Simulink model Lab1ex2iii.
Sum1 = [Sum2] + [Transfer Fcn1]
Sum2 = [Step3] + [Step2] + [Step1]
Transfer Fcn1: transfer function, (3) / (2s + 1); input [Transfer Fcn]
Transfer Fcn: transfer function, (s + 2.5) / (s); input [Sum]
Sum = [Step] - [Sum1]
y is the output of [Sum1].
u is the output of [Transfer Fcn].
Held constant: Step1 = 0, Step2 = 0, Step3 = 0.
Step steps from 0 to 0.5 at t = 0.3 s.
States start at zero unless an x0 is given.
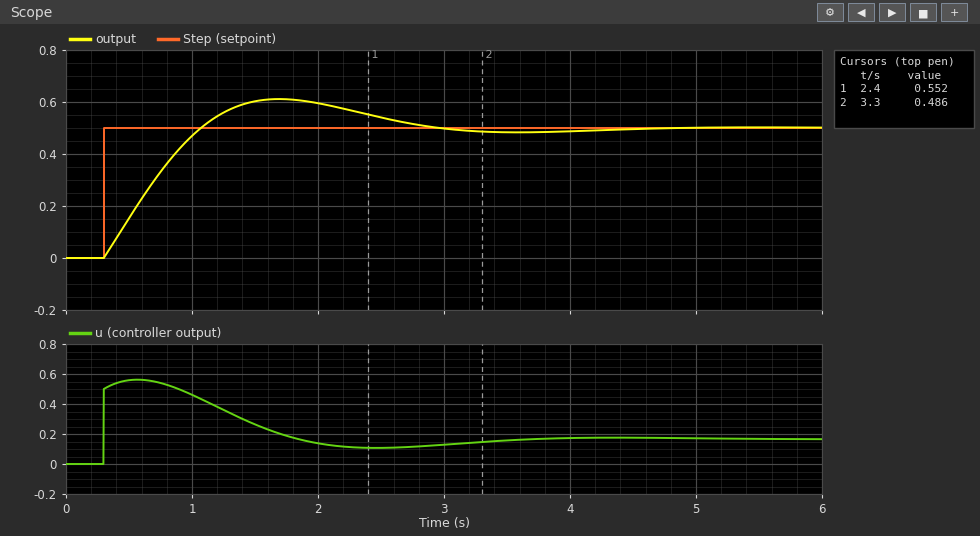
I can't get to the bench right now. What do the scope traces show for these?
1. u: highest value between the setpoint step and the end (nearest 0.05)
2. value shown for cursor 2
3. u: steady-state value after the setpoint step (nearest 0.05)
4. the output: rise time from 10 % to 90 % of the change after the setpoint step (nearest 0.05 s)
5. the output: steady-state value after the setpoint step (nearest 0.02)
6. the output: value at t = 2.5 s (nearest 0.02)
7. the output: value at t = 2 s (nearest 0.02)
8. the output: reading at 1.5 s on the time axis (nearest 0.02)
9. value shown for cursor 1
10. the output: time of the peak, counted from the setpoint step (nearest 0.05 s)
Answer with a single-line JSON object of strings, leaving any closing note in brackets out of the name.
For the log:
{"u: highest value between the setpoint step and the end": "0.55", "value shown for cursor 2": "0.486", "u: steady-state value after the setpoint step": "0.15", "the output: rise time from 10 % to 90 % of the change after the setpoint step": "0.60 s", "the output: steady-state value after the setpoint step": "0.50", "the output: value at t = 2.5 s": "0.54", "the output: value at t = 2 s": "0.60", "the output: reading at 1.5 s on the time axis": "0.60", "value shown for cursor 1": "0.552", "the output: time of the peak, counted from the setpoint step": "1.40 s"}
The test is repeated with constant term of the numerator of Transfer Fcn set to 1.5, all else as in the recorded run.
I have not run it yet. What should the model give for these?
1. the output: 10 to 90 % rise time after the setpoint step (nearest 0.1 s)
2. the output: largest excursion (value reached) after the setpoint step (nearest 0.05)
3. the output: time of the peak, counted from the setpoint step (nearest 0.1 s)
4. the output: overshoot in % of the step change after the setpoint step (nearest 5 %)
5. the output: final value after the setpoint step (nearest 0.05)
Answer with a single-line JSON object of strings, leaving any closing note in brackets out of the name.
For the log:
{"the output: 10 to 90 % rise time after the setpoint step": "0.8 s", "the output: largest excursion (value reached) after the setpoint step": "0.55", "the output: time of the peak, counted from the setpoint step": "1.8 s", "the output: overshoot in % of the step change after the setpoint step": "15 %", "the output: final value after the setpoint step": "0.50"}
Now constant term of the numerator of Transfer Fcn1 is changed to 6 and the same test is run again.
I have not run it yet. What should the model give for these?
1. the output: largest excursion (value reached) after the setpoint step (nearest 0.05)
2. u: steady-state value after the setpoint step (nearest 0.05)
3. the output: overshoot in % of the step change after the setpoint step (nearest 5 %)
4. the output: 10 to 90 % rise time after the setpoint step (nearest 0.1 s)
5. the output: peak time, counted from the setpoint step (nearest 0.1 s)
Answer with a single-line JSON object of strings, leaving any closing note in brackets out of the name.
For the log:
{"the output: largest excursion (value reached) after the setpoint step": "0.60", "u: steady-state value after the setpoint step": "0.10", "the output: overshoot in % of the step change after the setpoint step": "20 %", "the output: 10 to 90 % rise time after the setpoint step": "0.4 s", "the output: peak time, counted from the setpoint step": "0.9 s"}
